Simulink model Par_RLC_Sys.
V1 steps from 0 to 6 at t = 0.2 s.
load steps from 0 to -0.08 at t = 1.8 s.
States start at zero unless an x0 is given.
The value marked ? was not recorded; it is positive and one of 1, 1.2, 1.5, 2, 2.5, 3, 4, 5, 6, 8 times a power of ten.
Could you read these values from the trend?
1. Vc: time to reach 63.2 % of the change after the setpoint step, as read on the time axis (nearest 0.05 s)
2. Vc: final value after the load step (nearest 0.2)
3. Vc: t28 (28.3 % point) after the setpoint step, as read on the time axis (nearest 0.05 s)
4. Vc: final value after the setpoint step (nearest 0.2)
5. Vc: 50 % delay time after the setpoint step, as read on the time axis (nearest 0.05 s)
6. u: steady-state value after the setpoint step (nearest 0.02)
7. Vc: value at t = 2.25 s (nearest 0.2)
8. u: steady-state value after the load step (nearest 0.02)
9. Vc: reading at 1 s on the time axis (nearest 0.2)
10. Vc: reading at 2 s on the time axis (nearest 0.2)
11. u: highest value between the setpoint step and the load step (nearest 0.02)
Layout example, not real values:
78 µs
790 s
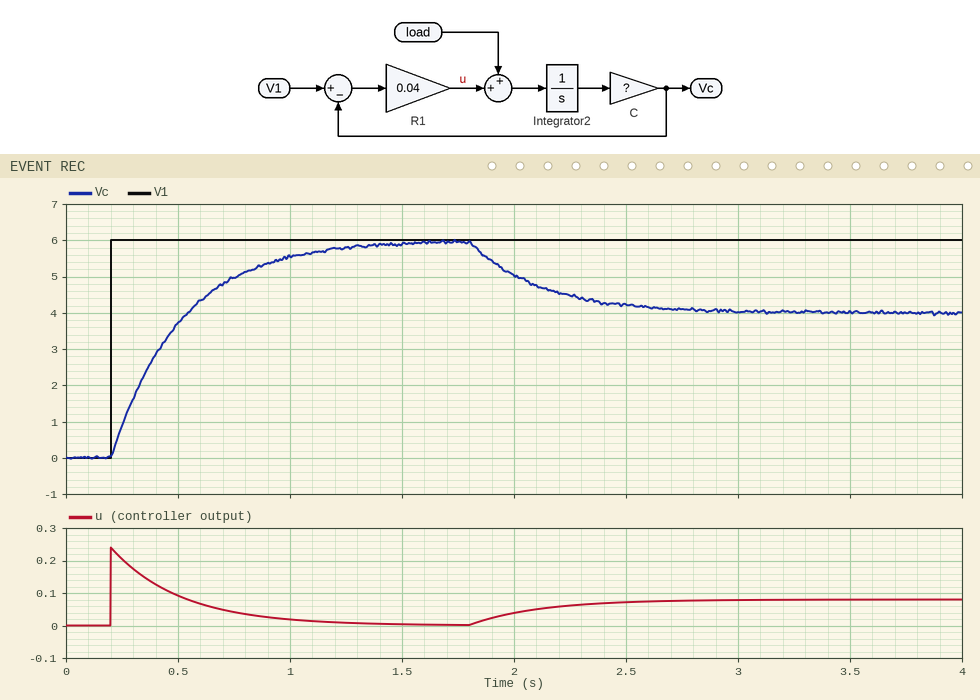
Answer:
0.50 s
4.0
0.30 s
6.0
0.40 s
0.00
4.4
0.08
5.6
5.0
0.24
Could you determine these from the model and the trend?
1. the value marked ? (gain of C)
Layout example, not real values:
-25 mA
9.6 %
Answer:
80
